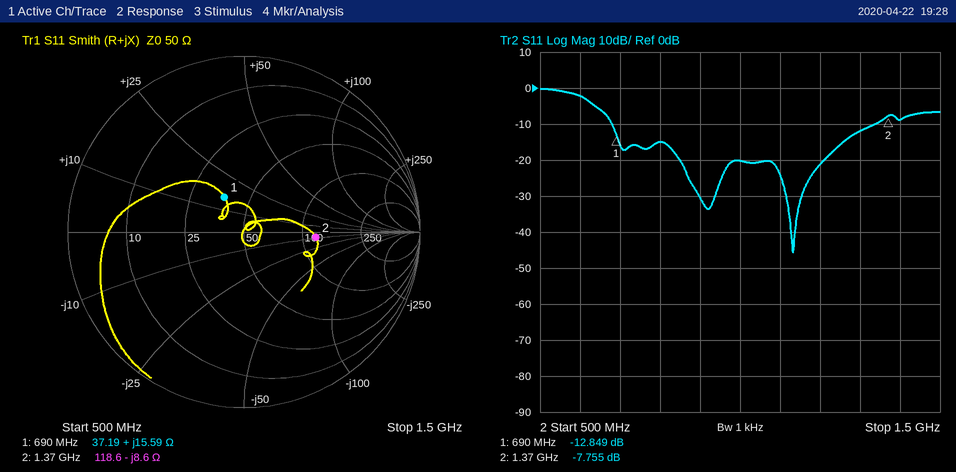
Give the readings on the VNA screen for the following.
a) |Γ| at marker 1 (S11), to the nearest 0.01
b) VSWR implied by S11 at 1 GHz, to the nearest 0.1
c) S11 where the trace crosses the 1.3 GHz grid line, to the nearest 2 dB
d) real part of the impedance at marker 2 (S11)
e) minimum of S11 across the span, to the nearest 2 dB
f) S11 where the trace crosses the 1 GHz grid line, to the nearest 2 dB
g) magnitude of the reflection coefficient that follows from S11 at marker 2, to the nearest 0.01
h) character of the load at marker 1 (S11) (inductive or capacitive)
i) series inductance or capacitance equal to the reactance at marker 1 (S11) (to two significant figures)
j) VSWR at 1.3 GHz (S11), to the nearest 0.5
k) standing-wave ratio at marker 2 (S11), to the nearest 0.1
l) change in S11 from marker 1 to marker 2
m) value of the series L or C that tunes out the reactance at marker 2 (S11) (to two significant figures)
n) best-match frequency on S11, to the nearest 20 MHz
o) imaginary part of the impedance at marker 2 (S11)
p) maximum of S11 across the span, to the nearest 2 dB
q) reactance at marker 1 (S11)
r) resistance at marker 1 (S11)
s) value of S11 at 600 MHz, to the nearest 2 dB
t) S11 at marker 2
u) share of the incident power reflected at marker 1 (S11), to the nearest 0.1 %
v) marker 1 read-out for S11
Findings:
0.23
1.2
-12 dB
118.6 Ω
-46 dB
-20 dB
0.41
inductive
3.6 nH
1.5
2.4
5.094 dB
1.0 nH
1.14 GHz
-8.6 Ω
0 dB
+15.59 Ω
37.19 Ω
-2 dB
-7.755 dB
5.2 %
-12.849 dB
